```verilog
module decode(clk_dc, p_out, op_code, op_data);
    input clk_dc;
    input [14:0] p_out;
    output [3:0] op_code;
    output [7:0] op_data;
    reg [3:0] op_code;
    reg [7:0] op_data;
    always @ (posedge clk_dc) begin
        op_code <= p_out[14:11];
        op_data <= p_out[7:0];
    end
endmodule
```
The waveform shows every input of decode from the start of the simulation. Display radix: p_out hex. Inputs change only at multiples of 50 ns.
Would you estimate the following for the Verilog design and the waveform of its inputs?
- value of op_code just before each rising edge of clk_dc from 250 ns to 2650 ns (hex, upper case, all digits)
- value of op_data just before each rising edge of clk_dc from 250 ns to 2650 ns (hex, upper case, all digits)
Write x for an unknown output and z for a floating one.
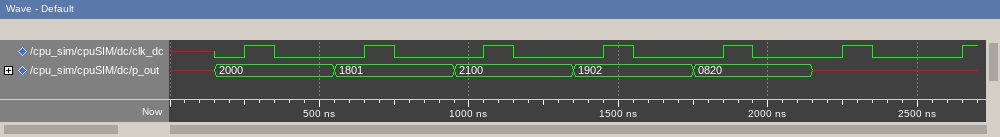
x, 4, 3, 4, 3, 1, x
x, 00, 01, 00, 02, 20, x
